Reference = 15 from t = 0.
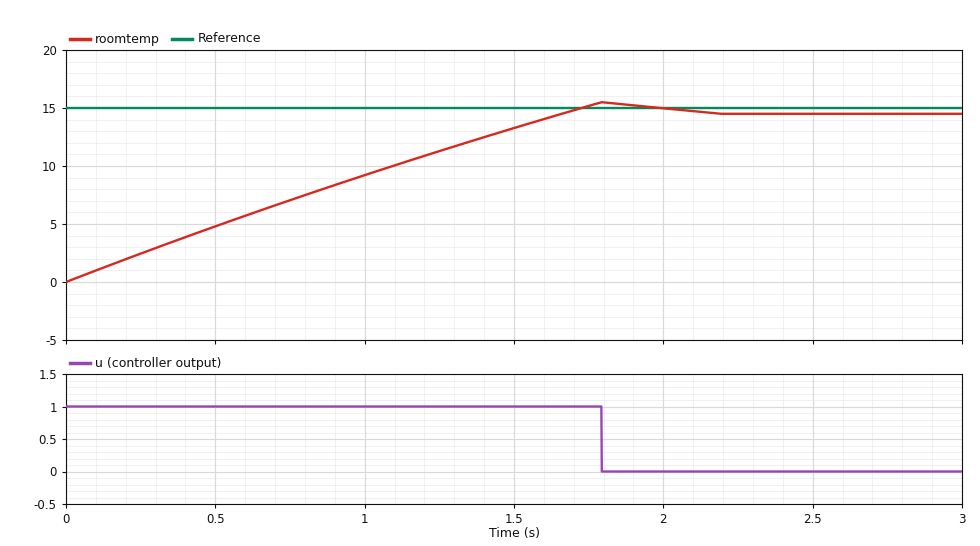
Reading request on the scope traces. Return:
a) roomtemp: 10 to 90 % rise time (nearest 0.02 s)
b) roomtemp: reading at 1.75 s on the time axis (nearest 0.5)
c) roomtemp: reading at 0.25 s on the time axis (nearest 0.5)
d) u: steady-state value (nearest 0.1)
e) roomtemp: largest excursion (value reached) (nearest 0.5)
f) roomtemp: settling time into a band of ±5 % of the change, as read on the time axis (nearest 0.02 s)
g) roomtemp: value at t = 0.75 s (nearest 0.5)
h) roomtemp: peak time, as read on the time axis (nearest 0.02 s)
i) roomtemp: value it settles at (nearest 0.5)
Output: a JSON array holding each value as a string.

["1.32 s", "15.0", "2.5", "0.0", "15.5", "1.90 s", "7.0", "1.80 s", "14.5"]
